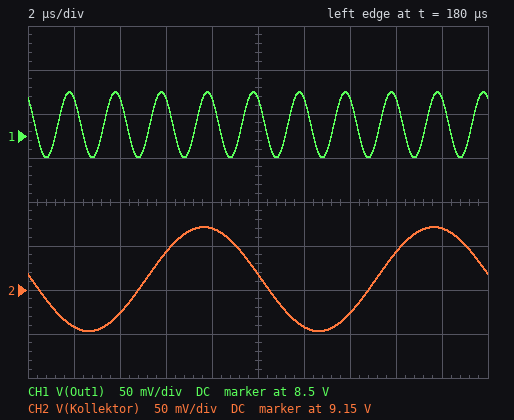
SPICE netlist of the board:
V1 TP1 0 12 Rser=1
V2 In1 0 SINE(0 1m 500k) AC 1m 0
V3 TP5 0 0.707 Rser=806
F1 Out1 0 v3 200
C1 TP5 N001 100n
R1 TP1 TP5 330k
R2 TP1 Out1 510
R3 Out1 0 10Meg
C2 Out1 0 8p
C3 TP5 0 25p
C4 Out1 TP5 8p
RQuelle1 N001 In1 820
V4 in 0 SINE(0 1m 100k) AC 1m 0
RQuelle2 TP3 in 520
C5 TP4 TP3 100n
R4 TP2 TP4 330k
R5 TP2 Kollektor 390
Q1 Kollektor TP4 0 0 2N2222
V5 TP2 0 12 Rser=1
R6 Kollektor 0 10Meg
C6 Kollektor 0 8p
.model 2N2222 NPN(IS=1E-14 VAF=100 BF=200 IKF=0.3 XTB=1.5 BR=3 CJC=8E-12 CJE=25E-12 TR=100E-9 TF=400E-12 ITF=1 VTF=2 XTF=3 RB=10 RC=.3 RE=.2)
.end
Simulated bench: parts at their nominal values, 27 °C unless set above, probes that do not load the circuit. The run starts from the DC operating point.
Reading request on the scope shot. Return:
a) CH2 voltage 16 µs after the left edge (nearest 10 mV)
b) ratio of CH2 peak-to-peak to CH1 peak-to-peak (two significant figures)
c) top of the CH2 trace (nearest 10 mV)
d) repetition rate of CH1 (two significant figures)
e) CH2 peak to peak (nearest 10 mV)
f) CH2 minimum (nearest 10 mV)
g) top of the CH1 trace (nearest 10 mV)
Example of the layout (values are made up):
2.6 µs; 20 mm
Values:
9.19 V; 1.6; 9.22 V; 500 kHz; 120 mV; 9.10 V; 8.55 V
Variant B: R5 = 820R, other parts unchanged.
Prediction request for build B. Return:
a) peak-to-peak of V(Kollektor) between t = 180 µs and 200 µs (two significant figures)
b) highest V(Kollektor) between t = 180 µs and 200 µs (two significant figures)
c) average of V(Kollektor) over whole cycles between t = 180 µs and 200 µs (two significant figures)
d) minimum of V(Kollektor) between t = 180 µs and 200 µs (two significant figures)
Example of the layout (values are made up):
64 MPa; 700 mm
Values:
230 mV; 6.3 V; 6.2 V; 6.1 V
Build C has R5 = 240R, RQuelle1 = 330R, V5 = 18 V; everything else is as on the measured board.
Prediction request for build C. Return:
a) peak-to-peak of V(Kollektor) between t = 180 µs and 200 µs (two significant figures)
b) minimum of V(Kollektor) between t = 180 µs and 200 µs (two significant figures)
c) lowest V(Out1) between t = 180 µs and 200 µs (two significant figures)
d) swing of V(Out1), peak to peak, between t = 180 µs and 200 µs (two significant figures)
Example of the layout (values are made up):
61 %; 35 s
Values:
94 mV; 15 V; 8.4 V; 140 mV
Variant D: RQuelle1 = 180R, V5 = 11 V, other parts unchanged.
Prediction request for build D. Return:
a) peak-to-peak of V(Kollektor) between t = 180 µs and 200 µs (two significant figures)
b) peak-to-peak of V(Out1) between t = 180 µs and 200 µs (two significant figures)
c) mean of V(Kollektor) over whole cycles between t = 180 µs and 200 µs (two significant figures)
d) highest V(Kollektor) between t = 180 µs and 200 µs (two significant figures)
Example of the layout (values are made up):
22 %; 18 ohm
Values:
110 mV; 180 mV; 8.4 V; 8.5 V
